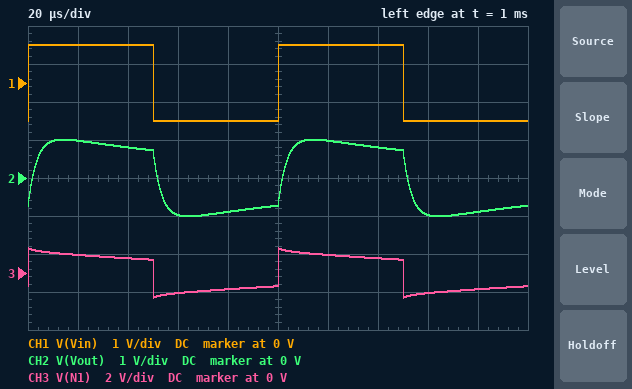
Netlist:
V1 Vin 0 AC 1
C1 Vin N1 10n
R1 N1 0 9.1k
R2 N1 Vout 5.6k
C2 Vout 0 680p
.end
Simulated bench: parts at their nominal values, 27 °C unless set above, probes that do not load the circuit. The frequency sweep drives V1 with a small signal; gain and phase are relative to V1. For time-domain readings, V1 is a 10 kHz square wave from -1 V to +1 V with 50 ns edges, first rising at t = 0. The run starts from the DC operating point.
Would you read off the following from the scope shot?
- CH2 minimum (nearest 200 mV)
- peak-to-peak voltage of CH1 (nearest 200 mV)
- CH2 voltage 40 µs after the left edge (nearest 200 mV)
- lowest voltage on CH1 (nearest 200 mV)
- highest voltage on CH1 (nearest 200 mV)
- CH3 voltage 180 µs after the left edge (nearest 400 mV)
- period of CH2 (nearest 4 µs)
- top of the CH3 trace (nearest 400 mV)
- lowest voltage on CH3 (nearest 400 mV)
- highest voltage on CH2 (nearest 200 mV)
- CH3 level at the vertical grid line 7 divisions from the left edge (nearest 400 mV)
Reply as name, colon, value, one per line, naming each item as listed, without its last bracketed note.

CH2 minimum: -1.0 V
peak-to-peak voltage of CH1: 2.0 V
CH2 voltage 40 µs after the left edge: 800 mV
lowest voltage on CH1: -1.0 V
highest voltage on CH1: 1.0 V
CH3 voltage 180 µs after the left edge: -800 mV
period of CH2: 100 µs
top of the CH3 trace: 1.2 V
lowest voltage on CH3: -1.2 V
highest voltage on CH2: 1.0 V
CH3 level at the vertical grid line 7 divisions from the left edge: 800 mV
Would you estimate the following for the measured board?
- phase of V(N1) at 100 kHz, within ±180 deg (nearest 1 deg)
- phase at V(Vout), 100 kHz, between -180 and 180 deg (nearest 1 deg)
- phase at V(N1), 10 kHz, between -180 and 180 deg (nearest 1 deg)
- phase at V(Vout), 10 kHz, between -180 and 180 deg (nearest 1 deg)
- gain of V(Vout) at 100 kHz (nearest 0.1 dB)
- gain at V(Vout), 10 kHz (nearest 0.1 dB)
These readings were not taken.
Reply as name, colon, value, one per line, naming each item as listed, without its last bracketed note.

phase of V(N1) at 100 kHz, within ±180 deg: 2 deg
phase at V(Vout), 100 kHz, between -180 and 180 deg: -65 deg
phase at V(N1), 10 kHz, between -180 and 180 deg: 10 deg
phase at V(Vout), 10 kHz, between -180 and 180 deg: -3 deg
gain of V(Vout) at 100 kHz: -8.4 dB
gain at V(Vout), 10 kHz: -0.9 dB
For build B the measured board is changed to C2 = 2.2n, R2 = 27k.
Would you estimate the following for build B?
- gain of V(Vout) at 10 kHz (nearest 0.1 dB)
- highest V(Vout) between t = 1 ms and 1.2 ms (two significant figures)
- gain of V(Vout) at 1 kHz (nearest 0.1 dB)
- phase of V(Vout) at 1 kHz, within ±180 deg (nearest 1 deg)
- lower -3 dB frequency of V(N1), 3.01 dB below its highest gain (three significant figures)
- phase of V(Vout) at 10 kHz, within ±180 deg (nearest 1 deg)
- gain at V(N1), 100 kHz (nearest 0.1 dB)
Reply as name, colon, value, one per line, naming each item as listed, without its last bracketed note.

gain of V(Vout) at 10 kHz: -12.1 dB
highest V(Vout) between t = 1 ms and 1.2 ms: 360 mV
gain of V(Vout) at 1 kHz: -7.3 dB
phase of V(Vout) at 1 kHz, within ±180 deg: 36 deg
lower -3 dB frequency of V(N1), 3.01 dB below its highest gain: 2.34 kHz
phase of V(Vout) at 10 kHz, within ±180 deg: -62 deg
gain at V(N1), 100 kHz: 0 dB
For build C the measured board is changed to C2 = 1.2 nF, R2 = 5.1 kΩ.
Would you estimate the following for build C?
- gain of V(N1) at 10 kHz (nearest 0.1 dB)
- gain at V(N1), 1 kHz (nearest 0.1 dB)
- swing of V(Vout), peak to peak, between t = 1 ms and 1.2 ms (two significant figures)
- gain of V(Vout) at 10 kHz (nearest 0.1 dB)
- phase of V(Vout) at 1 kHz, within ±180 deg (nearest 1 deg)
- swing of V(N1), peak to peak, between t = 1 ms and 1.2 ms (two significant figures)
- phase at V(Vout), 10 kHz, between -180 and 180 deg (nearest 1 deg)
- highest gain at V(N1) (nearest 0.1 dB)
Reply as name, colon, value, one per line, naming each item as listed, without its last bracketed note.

gain of V(N1) at 10 kHz: -1.0 dB
gain at V(N1), 1 kHz: -6.4 dB
swing of V(Vout), peak to peak, between t = 1 ms and 1.2 ms: 1.8 V
gain of V(Vout) at 10 kHz: -1.6 dB
phase of V(Vout) at 1 kHz, within ±180 deg: 55 deg
swing of V(N1), peak to peak, between t = 1 ms and 1.2 ms: 2.7 V
phase at V(Vout), 10 kHz, between -180 and 180 deg: -10 deg
highest gain at V(N1): 0 dB
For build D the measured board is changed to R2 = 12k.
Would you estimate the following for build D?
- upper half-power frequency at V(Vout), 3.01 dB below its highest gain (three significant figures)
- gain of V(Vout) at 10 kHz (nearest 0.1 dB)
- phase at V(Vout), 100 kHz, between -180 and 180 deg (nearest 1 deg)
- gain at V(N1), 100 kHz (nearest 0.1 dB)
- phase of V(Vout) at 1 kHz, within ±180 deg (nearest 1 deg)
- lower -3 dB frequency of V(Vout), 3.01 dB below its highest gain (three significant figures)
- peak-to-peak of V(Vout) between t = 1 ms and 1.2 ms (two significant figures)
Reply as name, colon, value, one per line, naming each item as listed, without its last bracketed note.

upper half-power frequency at V(Vout), 3.01 dB below its highest gain: 24.0 kHz
gain of V(Vout) at 10 kHz: -1.6 dB
phase at V(Vout), 100 kHz, between -180 and 180 deg: -77 deg
gain at V(N1), 100 kHz: 0 dB
phase of V(Vout) at 1 kHz, within ±180 deg: 56 deg
lower -3 dB frequency of V(Vout), 3.01 dB below its highest gain: 1.42 kHz
peak-to-peak of V(Vout) between t = 1 ms and 1.2 ms: 1.8 V
